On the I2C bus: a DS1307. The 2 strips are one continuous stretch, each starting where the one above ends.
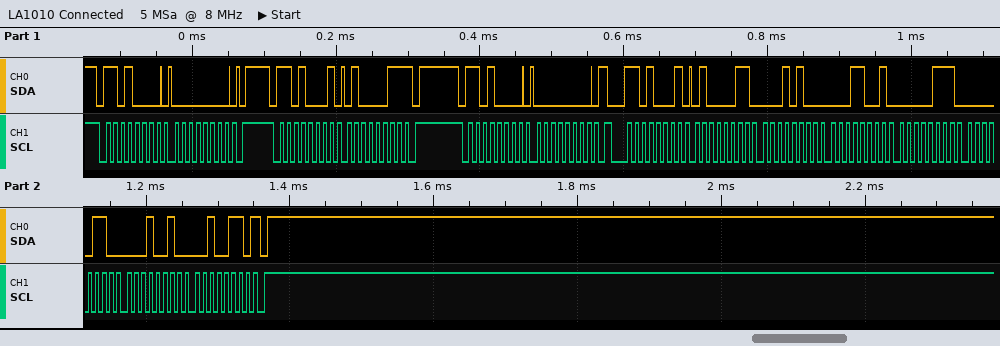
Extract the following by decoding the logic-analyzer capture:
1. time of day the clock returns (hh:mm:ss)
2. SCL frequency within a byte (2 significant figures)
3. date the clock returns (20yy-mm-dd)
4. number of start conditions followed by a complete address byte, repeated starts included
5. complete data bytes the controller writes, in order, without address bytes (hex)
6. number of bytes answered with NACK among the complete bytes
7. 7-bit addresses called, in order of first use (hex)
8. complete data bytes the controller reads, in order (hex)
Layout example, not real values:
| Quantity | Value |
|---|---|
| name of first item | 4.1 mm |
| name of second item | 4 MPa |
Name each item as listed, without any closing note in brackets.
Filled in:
| Quantity | Value |
|---|---|
| time of day the clock returns | 19:14:43 |
| SCL frequency within a byte | 100 kHz |
| date the clock returns | 2026-12-06 |
| number of start conditions followed by a complete address byte, repeated starts included | 4 |
| complete data bytes the controller writes, in order, without address bytes | 00 00 |
| number of bytes answered with NACK among the complete bytes | 2 |
| 7-bit addresses called, in order of first use | 0x68 |
| complete data bytes the controller reads, in order | 43 43 14 19 07 06 12 26 |
